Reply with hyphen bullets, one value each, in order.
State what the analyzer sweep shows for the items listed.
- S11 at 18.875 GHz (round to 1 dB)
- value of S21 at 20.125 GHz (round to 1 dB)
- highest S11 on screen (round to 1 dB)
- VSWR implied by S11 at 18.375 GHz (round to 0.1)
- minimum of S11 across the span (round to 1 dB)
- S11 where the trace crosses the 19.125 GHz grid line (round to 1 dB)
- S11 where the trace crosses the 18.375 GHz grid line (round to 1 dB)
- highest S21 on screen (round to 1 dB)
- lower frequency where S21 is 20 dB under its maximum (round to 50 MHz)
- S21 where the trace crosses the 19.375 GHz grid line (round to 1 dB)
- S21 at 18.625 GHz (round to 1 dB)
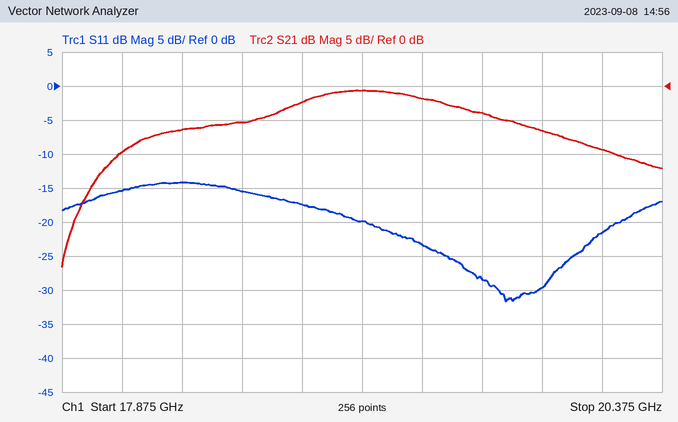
- -17 dB
- -9 dB
- -14 dB
- 1.5
- -32 dB
- -20 dB
- -14 dB
- -1 dB
- 17.90 GHz
- -2 dB
- -5 dB
